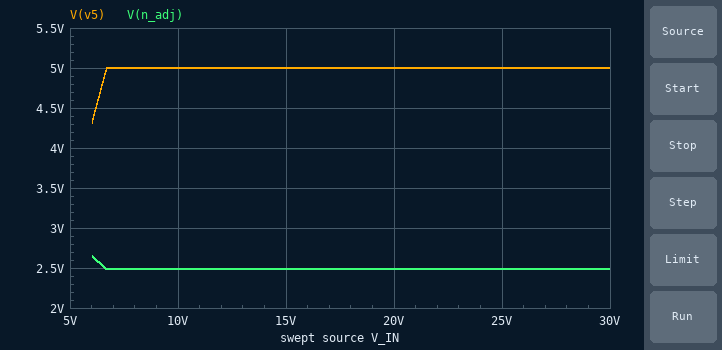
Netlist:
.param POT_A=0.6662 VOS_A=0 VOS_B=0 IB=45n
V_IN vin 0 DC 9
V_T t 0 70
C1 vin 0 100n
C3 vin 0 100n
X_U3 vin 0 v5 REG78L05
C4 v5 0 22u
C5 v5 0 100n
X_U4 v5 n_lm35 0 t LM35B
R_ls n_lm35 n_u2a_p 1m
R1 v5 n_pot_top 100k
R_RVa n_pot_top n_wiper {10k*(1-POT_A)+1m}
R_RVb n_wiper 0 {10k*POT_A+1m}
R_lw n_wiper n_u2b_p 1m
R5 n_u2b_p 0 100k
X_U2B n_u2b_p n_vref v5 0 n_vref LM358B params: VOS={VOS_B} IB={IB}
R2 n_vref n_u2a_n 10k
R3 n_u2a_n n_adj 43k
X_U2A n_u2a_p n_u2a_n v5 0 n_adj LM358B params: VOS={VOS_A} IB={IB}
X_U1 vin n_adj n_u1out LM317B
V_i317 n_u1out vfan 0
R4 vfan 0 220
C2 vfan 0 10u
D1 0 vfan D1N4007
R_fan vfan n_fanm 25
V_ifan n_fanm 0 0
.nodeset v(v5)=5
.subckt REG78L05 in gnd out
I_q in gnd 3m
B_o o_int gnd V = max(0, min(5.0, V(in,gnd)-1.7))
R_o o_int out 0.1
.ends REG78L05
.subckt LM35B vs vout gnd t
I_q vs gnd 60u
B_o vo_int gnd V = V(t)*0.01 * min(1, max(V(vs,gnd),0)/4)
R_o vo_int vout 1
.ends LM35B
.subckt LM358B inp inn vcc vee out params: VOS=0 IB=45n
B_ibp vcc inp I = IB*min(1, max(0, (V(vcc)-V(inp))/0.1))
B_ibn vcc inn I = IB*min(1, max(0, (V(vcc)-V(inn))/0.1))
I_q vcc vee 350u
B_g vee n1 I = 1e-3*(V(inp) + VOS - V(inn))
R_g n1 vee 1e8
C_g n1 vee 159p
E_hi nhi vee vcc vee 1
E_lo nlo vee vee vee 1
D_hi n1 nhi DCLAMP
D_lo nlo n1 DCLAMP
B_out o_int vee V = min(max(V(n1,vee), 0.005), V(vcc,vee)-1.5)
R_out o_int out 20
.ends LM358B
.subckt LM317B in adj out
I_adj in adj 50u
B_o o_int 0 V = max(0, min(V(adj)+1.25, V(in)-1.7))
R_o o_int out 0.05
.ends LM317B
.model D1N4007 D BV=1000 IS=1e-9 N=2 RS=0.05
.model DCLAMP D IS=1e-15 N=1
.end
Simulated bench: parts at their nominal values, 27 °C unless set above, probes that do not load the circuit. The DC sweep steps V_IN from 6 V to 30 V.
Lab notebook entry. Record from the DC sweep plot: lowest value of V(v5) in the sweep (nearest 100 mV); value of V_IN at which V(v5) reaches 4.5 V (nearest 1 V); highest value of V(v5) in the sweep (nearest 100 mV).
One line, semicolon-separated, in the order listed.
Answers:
4.3 V; 6 V; 5.0 V
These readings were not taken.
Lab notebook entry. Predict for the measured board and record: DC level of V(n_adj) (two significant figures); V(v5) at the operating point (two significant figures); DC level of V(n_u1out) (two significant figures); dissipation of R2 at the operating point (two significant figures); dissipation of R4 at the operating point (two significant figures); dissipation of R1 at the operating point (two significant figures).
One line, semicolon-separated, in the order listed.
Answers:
2.5 V; 5.0 V; 3.7 V; 17 µW; 63 mW; 210 µW
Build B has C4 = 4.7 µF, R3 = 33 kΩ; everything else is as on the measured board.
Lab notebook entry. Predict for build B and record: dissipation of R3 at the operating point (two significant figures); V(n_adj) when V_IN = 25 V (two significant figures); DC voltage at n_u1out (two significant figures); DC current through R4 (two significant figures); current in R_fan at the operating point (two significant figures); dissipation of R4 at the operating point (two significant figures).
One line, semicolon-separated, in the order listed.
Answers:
57 µW; 2.1 V; 3.3 V; 15 mA; 130 mA; 50 mW
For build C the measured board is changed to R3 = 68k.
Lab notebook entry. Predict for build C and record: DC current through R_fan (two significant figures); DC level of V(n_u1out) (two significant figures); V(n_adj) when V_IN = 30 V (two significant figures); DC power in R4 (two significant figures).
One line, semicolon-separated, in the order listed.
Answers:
190 mA; 4.7 V; 3.5 V; 100 mW
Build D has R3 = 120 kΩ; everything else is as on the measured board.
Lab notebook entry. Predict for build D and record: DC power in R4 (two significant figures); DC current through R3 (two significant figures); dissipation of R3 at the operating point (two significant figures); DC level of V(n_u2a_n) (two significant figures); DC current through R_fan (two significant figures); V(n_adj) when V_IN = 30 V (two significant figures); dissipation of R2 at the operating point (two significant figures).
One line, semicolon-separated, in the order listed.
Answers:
100 mW; 25 µA; 73 µW; 530 mV; 190 mA; 3.5 V; 6.1 µW
